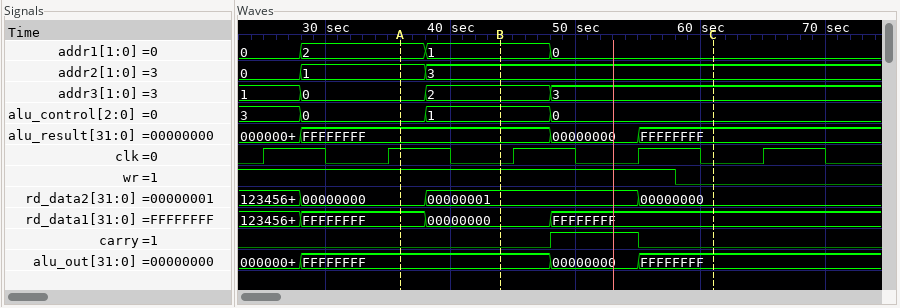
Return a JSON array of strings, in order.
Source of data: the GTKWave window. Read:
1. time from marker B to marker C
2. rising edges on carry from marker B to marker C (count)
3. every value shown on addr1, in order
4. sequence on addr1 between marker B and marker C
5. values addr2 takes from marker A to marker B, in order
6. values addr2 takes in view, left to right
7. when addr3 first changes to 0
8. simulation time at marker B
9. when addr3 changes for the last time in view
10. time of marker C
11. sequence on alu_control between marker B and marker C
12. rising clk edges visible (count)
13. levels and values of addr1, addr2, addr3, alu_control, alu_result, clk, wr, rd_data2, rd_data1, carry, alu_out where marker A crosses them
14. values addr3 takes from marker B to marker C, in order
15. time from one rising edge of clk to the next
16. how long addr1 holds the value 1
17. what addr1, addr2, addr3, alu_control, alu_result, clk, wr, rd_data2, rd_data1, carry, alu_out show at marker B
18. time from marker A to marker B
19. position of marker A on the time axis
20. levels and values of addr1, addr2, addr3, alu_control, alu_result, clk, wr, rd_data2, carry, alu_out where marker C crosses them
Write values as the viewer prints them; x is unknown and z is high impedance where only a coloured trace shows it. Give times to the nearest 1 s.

["17 s", "1", "0, 2, 1, 0", "1, 0", "1, 3", "0, 1, 3", "28 s", "44 s", "48 s", "61 s", "1, 0", "5", "addr1=2, addr2=1, addr3=0, alu_control=0, alu_result=FFFFFFFF, clk=1, wr=1, rd_data2=00000000, rd_data1=FFFFFFFF, carry=0, alu_out=FFFFFFFF", "2, 3", "10 s", "10 s", "addr1=1, addr2=3, addr3=2, alu_control=1, alu_result=FFFFFFFF, clk=0, wr=1, rd_data2=00000001, rd_data1=00000000, carry=0, alu_out=FFFFFFFF", "8 s", "36 s", "addr1=0, addr2=3, addr3=3, alu_control=0, alu_result=FFFFFFFF, clk=0, wr=0, rd_data2=00000000, carry=0, alu_out=FFFFFFFF"]
